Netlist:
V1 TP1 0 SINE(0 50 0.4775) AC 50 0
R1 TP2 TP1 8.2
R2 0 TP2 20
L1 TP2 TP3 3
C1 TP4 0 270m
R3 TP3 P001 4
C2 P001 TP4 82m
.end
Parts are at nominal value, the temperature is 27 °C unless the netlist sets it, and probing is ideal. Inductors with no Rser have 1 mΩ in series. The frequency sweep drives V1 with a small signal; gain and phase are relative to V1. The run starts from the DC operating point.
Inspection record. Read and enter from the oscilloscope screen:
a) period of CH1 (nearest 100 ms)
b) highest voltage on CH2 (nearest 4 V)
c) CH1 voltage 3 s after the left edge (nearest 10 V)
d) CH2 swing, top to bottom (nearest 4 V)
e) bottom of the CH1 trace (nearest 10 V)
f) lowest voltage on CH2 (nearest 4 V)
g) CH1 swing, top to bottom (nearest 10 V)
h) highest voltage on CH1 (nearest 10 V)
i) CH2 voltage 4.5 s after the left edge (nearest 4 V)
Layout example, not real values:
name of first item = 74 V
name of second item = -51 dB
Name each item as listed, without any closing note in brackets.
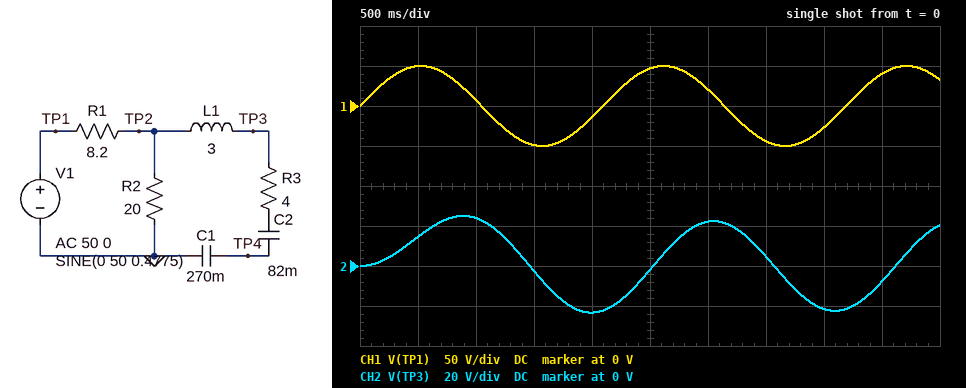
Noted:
period of CH1 = 2.1 s
highest voltage on CH2 = 24 V
CH1 voltage 3 s after the left edge = 20 V
CH2 swing, top to bottom = 48 V
bottom of the CH1 trace = -50 V
lowest voltage on CH2 = -24 V
CH1 swing, top to bottom = 100 V
highest voltage on CH1 = 50 V
CH2 voltage 4.5 s after the left edge = -8 V
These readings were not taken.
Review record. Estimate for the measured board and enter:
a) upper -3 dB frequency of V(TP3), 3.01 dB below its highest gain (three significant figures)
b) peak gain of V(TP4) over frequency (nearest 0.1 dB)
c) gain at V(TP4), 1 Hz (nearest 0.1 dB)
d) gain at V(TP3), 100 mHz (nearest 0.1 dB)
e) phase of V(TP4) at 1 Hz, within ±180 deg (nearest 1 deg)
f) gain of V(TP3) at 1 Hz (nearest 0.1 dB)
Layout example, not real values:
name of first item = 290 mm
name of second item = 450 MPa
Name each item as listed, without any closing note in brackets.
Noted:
upper -3 dB frequency of V(TP3), 3.01 dB below its highest gain = 425 mHz
peak gain of V(TP4) over frequency = -15.6 dB
gain at V(TP4), 1 Hz = -33.2 dB
gain at V(TP3), 100 mHz = -2.9 dB
phase of V(TP4) at 1 Hz, within ±180 deg = -149 deg
gain of V(TP3) at 1 Hz = -15.1 dB
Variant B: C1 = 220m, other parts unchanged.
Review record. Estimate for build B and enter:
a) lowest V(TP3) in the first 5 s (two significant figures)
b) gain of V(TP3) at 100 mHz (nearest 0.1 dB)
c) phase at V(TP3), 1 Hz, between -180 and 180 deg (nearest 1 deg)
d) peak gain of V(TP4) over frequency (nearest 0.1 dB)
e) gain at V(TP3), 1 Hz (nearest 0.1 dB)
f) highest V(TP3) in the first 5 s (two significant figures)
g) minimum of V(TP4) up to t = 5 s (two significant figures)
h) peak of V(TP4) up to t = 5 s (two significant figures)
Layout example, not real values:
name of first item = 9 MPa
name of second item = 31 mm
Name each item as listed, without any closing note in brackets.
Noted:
lowest V(TP3) in the first 5 s = -24 V
gain of V(TP3) at 100 mHz = -2.9 dB
phase at V(TP3), 1 Hz, between -180 and 180 deg = -92 deg
peak gain of V(TP4) over frequency = -14.3 dB
gain at V(TP3), 1 Hz = -14.9 dB
highest V(TP3) in the first 5 s = 26 V
minimum of V(TP4) up to t = 5 s = -5.4 V
peak of V(TP4) up to t = 5 s = 6.1 V
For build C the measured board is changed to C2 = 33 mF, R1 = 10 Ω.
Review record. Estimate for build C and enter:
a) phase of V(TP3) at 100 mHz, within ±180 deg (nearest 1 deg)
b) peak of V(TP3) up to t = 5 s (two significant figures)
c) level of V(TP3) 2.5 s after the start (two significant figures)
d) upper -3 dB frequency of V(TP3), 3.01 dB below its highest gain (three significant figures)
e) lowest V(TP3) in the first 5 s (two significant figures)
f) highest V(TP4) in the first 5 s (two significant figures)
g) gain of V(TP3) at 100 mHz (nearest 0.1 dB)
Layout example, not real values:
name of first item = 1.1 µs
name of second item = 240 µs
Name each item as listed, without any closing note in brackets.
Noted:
phase of V(TP3) at 100 mHz, within ±180 deg = -7 deg
peak of V(TP3) up to t = 5 s = 37 V
level of V(TP3) 2.5 s after the start = 7.6 V
upper -3 dB frequency of V(TP3), 3.01 dB below its highest gain = 648 mHz
lowest V(TP3) in the first 5 s = -37 V
highest V(TP4) in the first 5 s = 3.8 V
gain of V(TP3) at 100 mHz = -3.4 dB
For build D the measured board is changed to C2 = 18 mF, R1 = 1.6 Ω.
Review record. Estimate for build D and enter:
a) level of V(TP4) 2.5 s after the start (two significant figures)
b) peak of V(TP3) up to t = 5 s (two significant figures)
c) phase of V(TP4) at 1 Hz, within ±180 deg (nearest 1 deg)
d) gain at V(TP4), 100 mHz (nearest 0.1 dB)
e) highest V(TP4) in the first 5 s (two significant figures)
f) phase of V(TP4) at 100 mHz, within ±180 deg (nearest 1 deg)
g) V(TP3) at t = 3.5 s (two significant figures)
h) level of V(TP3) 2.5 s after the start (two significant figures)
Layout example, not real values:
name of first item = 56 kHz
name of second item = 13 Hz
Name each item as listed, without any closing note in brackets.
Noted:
level of V(TP4) 2.5 s after the start = 3.4 V
peak of V(TP3) up to t = 5 s = 81 V
phase of V(TP4) at 1 Hz, within ±180 deg = -150 deg
gain at V(TP4), 100 mHz = -24.6 dB
highest V(TP4) in the first 5 s = 5.0 V
phase of V(TP4) at 100 mHz, within ±180 deg = -3 deg
V(TP3) at t = 3.5 s = -57 V
level of V(TP3) 2.5 s after the start = 67 V
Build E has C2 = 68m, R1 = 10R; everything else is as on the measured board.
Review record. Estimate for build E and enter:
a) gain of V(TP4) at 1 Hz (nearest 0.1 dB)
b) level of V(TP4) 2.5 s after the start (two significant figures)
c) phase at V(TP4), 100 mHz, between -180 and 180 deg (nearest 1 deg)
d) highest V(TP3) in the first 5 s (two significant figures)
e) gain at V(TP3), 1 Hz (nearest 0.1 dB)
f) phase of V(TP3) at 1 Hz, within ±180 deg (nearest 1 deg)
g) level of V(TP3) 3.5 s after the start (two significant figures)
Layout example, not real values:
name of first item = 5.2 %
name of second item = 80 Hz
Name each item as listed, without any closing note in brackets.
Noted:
gain of V(TP4) at 1 Hz = -33.8 dB
level of V(TP4) 2.5 s after the start = -2.2 V
phase at V(TP4), 100 mHz, between -180 and 180 deg = -21 deg
highest V(TP3) in the first 5 s = 24 V
gain at V(TP3), 1 Hz = -15.3 dB
phase of V(TP3) at 1 Hz, within ±180 deg = -92 deg
level of V(TP3) 3.5 s after the start = 4.0 V
